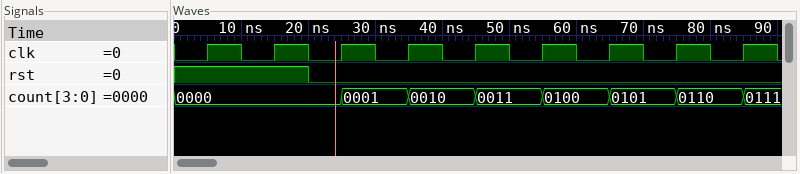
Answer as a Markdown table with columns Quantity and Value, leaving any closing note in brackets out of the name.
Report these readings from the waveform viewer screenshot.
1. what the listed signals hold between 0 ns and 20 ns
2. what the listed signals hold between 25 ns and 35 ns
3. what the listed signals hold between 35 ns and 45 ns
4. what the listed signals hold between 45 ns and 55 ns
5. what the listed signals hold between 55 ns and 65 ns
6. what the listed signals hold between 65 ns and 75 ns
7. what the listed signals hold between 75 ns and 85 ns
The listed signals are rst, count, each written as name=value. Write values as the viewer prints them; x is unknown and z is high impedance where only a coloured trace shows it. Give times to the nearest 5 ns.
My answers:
| Quantity | Value |
|---|---|
| what the listed signals hold between 0 ns and 20 ns | rst=1, count=0000 |
| what the listed signals hold between 25 ns and 35 ns | rst=0, count=0001 |
| what the listed signals hold between 35 ns and 45 ns | rst=0, count=0010 |
| what the listed signals hold between 45 ns and 55 ns | rst=0, count=0011 |
| what the listed signals hold between 55 ns and 65 ns | rst=0, count=0100 |
| what the listed signals hold between 65 ns and 75 ns | rst=0, count=0101 |
| what the listed signals hold between 75 ns and 85 ns | rst=0, count=0110 |
